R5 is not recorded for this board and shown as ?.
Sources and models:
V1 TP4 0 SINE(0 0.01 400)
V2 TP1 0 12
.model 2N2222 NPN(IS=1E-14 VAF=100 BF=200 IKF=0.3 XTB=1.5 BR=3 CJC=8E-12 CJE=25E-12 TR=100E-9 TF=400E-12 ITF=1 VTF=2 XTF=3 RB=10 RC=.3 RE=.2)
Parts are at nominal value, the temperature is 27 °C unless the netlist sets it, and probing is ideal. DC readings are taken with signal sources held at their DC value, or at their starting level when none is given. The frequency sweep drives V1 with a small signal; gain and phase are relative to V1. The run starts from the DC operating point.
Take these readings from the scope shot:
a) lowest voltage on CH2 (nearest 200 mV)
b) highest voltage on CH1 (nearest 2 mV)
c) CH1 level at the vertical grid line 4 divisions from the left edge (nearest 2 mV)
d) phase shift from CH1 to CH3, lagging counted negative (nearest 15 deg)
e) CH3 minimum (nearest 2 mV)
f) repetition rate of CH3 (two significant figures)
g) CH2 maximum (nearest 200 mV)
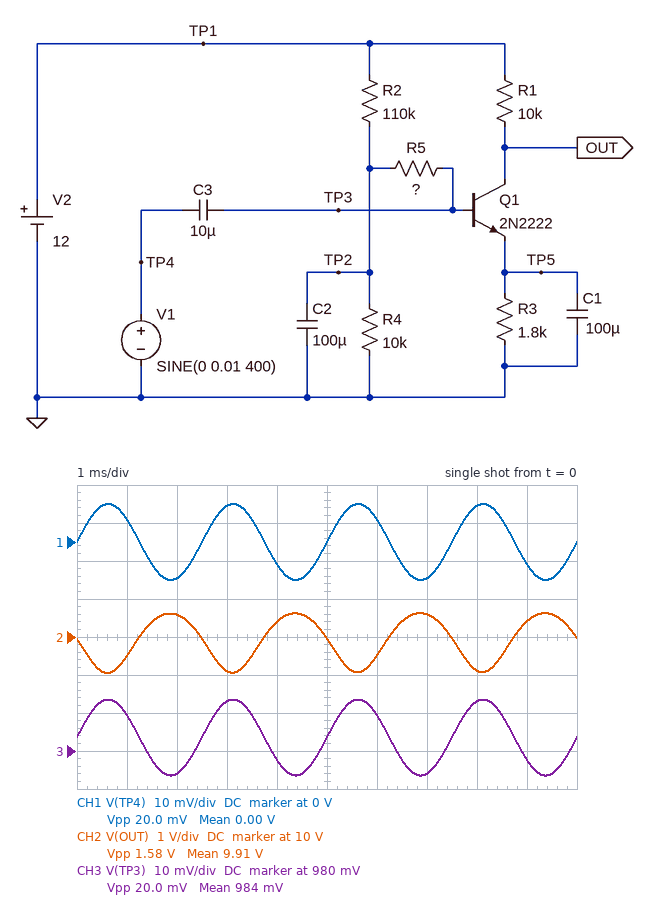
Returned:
9.0 V
10 mV
-6 mV
0 deg
974 mV
400 Hz
10.6 V
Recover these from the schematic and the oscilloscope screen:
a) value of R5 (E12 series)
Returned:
8.2 kΩ
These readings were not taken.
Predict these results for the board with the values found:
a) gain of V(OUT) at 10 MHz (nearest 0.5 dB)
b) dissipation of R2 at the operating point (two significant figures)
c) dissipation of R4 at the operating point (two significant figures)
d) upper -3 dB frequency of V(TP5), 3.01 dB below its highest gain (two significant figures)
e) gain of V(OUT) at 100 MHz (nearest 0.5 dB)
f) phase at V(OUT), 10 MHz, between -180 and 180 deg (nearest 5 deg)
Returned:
30.0 dB
1.1 mW
98 µW
18 Hz
10.5 dB
110 deg
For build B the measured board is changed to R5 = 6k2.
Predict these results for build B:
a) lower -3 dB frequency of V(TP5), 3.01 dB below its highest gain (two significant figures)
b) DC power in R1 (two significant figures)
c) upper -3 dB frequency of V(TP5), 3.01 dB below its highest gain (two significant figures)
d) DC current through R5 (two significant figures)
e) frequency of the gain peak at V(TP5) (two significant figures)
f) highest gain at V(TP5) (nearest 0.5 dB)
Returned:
2.0 Hz
430 µW
19 Hz
950 nA
6.2 Hz
-2.5 dB
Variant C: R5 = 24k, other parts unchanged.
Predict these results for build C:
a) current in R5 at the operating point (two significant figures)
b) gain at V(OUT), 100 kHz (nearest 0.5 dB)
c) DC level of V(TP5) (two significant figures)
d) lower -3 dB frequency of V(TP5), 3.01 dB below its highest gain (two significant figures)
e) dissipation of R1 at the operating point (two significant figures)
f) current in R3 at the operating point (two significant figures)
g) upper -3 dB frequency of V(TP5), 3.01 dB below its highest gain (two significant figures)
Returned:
910 nA
37.5 dB
360 mV
640 mHz
390 µW
200 µA
15 Hz
